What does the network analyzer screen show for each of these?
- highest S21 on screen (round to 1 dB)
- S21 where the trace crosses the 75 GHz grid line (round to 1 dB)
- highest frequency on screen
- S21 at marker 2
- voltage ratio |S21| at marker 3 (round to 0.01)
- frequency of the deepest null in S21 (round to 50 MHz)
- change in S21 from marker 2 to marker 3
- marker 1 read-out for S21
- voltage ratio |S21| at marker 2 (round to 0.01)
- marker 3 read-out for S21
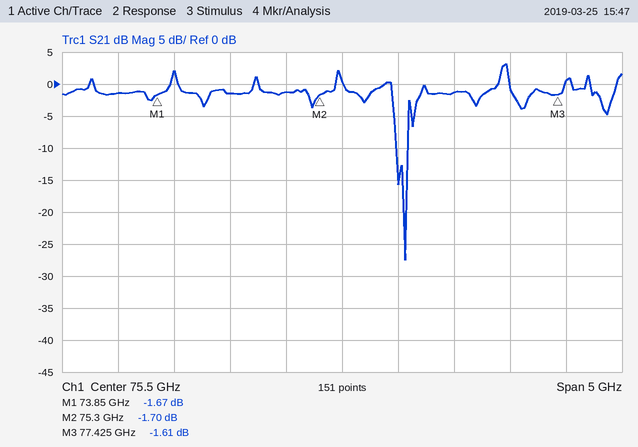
3 dB
-1 dB
78 GHz
-1.70 dB
0.83
76.05 GHz
0.09 dB
-1.67 dB
0.82
-1.61 dB
